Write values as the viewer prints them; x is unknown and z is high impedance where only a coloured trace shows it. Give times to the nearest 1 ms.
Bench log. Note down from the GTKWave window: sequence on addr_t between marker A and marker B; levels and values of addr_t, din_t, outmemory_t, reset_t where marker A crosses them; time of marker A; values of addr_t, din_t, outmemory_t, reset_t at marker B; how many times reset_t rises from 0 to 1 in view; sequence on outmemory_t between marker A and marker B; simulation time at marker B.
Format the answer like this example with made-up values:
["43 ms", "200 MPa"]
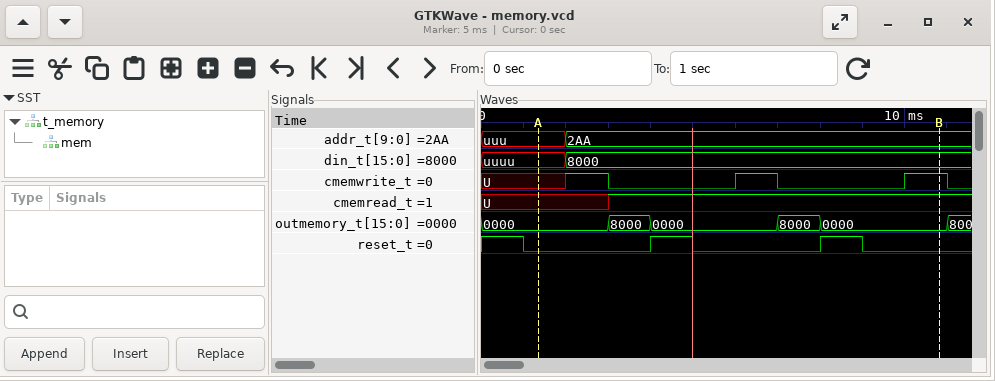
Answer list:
["uuu, 2AA", "addr_t=uuu, din_t=uuuu, outmemory_t=0000, reset_t=0", "1 ms", "addr_t=2AA, din_t=8000, outmemory_t=0000, reset_t=0", "2", "0000, 8000, 0000, 8000, 0000", "11 ms"]
